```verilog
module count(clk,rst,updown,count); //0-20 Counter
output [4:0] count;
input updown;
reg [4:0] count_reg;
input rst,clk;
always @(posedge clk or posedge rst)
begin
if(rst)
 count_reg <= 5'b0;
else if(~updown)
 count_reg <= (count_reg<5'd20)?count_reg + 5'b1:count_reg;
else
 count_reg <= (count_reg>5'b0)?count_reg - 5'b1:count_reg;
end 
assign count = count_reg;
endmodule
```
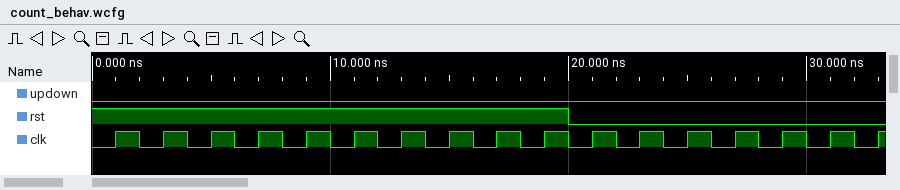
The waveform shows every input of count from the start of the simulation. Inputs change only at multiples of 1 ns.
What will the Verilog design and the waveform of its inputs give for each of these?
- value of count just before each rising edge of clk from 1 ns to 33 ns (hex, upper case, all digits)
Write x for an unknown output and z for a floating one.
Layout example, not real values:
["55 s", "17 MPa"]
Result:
["00, 00, 00, 00, 00, 00, 00, 00, 00, 00, 00, 01, 02, 03, 04, 05, 06"]
